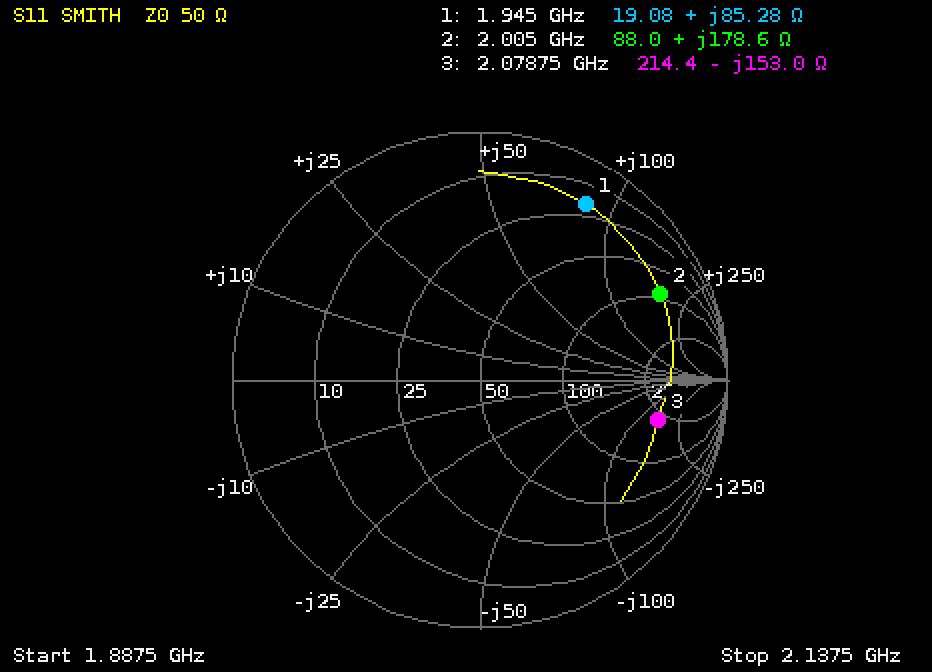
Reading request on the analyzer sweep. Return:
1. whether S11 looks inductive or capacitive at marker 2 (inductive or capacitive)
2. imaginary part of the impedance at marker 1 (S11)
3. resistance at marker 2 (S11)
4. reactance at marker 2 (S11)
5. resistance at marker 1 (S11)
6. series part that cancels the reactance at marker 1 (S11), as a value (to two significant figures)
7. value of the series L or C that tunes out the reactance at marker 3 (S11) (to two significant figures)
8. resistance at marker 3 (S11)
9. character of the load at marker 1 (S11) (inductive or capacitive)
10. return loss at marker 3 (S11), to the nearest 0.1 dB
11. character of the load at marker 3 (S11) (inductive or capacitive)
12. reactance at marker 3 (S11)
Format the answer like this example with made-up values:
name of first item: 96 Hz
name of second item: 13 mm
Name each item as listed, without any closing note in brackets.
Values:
whether S11 looks inductive or capacitive at marker 2: inductive
imaginary part of the impedance at marker 1: +85.28 Ω
resistance at marker 2: 88.0 Ω
reactance at marker 2: +178.6 Ω
resistance at marker 1: 19.08 Ω
series part that cancels the reactance at marker 1 (S11), as a value: 960 fF
value of the series L or C that tunes out the reactance at marker 3 (S11): 12 nH
resistance at marker 3: 214.4 Ω
character of the load at marker 1 (S11): inductive
return loss at marker 3 (S11), to the nearest 0.1 dB: 2.7 dB
character of the load at marker 3 (S11): capacitive
reactance at marker 3: -153.0 Ω
